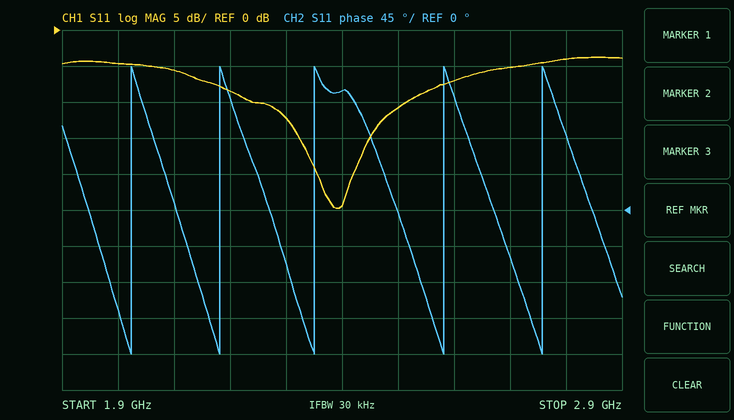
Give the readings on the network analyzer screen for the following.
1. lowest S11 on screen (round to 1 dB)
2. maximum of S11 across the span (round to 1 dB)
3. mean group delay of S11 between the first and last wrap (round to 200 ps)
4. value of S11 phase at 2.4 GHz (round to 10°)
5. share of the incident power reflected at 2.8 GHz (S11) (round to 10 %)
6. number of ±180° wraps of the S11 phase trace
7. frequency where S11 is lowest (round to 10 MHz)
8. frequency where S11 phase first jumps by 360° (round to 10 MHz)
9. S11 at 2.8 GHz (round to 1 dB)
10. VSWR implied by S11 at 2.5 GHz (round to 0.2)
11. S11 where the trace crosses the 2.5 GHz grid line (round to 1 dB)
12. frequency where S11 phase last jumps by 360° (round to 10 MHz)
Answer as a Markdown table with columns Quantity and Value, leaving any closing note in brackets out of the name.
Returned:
| Quantity | Value |
|---|---|
| lowest S11 on screen | -25 dB |
| maximum of S11 across the span | -4 dB |
| mean group delay of S11 between the first and last wrap | 5.4 ns |
| value of S11 phase at 2.4 GHz | 150° |
| share of the incident power reflected at 2.8 GHz (S11) | 40 % |
| number of ±180° wraps of the S11 phase trace | 5 |
| frequency where S11 is lowest | 2.39 GHz |
| frequency where S11 phase first jumps by 360° | 2.02 GHz |
| S11 at 2.8 GHz | -4 dB |
| VSWR implied by S11 at 2.5 GHz | 1.8 |
| S11 where the trace crosses the 2.5 GHz grid line | -11 dB |
| frequency where S11 phase last jumps by 360° | 2.76 GHz |
